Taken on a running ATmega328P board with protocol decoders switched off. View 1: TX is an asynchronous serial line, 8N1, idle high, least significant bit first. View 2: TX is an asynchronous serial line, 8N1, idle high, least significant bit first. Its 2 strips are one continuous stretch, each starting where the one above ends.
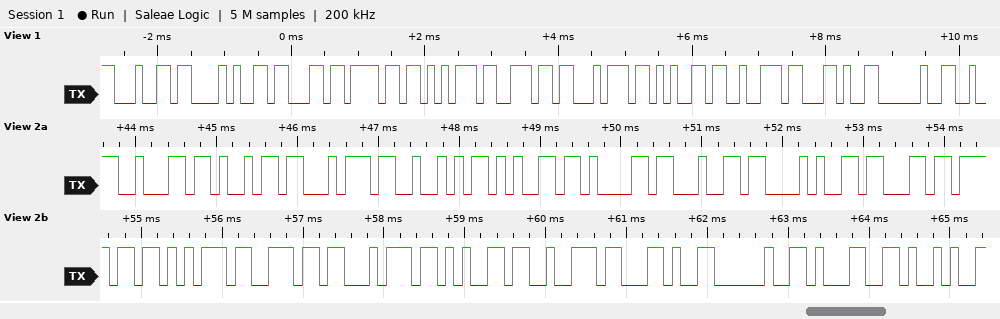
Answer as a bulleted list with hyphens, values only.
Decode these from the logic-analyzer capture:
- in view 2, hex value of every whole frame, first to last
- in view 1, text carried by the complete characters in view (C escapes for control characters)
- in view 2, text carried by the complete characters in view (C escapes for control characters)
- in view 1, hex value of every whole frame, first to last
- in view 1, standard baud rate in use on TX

- 62 69 74 52 65 61 64 28 63 6F 75 6E 74 65 72 2C 20 31 29
- "d(counter, "
- "bitRead(counter, 1)"
- 64 28 63 6F 75 6E 74 65 72 2C 20
- 9600 baud
